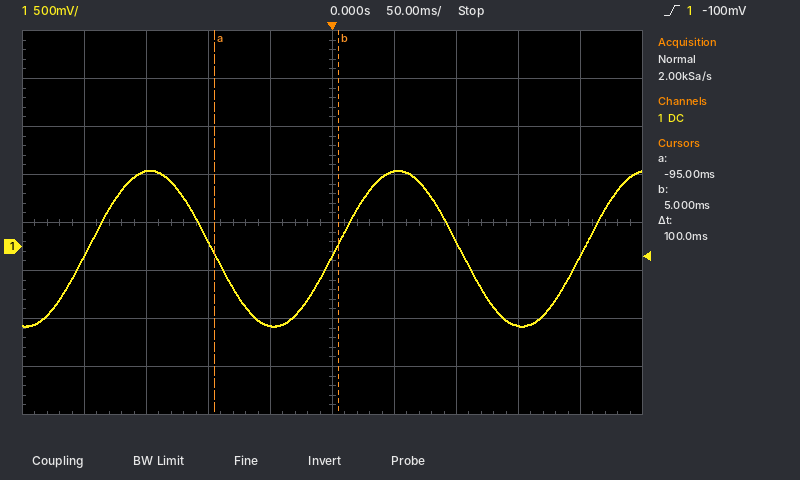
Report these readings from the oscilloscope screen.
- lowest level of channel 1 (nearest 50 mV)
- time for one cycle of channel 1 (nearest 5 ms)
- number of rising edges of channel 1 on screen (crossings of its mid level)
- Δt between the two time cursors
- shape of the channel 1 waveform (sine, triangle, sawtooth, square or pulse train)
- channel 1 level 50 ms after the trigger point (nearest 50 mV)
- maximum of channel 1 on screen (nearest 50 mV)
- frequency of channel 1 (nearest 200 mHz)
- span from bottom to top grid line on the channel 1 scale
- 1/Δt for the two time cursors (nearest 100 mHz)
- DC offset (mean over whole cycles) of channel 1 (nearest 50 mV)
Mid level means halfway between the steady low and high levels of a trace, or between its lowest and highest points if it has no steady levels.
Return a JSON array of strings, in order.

["-850 mV", "200 ms", "3", "100 ms", "sine", "800 mV", "800 mV", "5.0 Hz", "4 V", "10.0 Hz", "0 mV"]
